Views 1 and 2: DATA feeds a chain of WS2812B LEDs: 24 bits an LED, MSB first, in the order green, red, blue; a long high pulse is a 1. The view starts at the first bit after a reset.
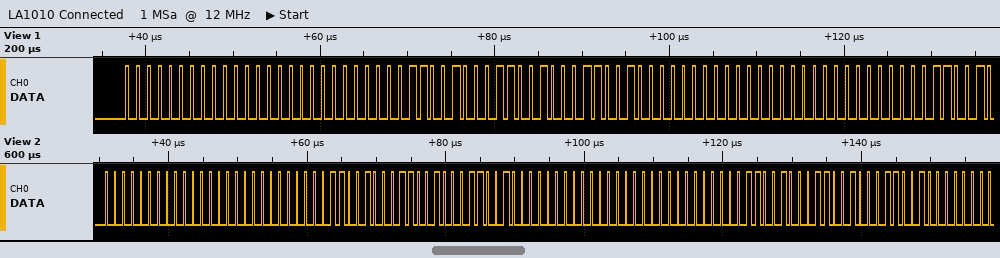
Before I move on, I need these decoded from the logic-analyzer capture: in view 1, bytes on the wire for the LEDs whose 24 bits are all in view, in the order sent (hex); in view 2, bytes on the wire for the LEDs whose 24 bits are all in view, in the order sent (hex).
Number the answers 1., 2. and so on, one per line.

1. 00 00 00 32 32 32 00 00 00
2. 00 00 00 32 32 32 00 00 00 32 32 32
